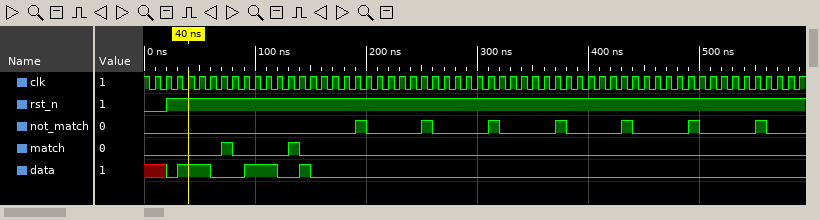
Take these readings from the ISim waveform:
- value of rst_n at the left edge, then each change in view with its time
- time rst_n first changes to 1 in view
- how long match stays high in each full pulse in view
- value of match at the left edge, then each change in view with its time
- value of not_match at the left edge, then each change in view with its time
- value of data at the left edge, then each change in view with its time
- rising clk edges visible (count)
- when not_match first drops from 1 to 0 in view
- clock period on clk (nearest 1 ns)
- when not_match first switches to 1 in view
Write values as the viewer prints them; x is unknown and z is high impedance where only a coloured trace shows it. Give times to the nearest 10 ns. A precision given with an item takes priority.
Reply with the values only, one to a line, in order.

0, 1 at 20 ns
20 ns
10 ns, 10 ns
0, 1 at 70 ns, 0 at 80 ns, 1 at 130 ns, 0 at 140 ns
0, 1 at 190 ns, 0 at 200 ns, 1 at 250 ns, 0 at 260 ns, 1 at 310 ns, 0 at 320 ns, 1 at 370 ns, 0 at 380 ns, 1 at 430 ns, 0 at 440 ns, 1 at 490 ns, 0 at 500 ns, 1 at 550 ns, 0 at 560 ns
x, 0 at 20 ns, 1 at 30 ns, 0 at 60 ns, 1 at 90 ns, 0 at 120 ns, 1 at 140 ns, 0 at 150 ns
59
200 ns
10 ns
190 ns
